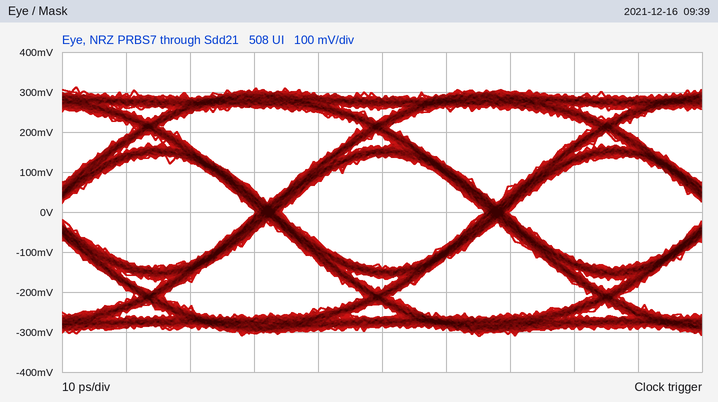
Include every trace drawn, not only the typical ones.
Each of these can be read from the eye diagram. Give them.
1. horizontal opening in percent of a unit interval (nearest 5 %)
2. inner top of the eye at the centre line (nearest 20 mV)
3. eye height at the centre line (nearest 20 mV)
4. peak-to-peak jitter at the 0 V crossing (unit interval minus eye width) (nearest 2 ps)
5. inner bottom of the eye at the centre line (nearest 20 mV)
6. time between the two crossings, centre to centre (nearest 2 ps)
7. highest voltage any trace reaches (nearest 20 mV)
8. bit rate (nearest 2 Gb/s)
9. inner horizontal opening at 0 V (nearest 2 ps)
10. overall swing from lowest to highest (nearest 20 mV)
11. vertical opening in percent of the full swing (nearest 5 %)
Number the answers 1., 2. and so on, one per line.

1. 90 %
2. 140 mV
3. 280 mV
4. 4 ps
5. -140 mV
6. 36 ps
7. 320 mV
8. 28 Gb/s
9. 32 ps
10. 620 mV
11. 45 %
